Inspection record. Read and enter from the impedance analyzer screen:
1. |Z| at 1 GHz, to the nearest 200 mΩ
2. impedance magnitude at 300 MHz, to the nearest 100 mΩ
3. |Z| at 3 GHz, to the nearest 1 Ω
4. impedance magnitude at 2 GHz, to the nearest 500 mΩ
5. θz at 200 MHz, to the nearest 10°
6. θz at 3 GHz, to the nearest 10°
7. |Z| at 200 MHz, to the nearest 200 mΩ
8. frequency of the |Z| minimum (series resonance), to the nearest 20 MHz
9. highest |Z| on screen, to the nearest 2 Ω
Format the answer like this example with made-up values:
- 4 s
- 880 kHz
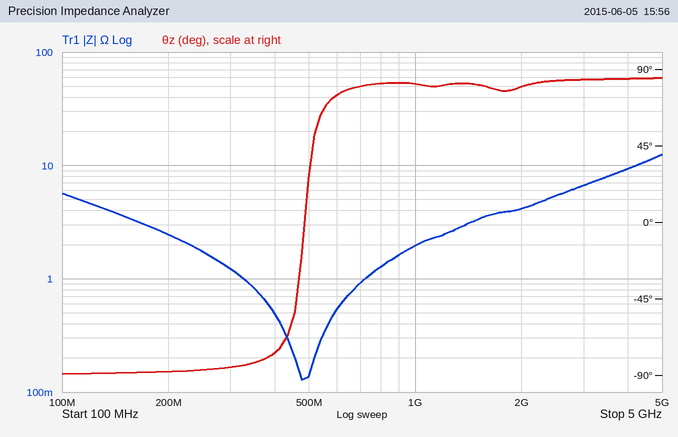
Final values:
- 2.0 Ω
- 1.2 Ω
- 7 Ω
- 4.0 Ω
- -90°
- 80°
- 2.4 Ω
- 480 MHz
- 12 Ω
